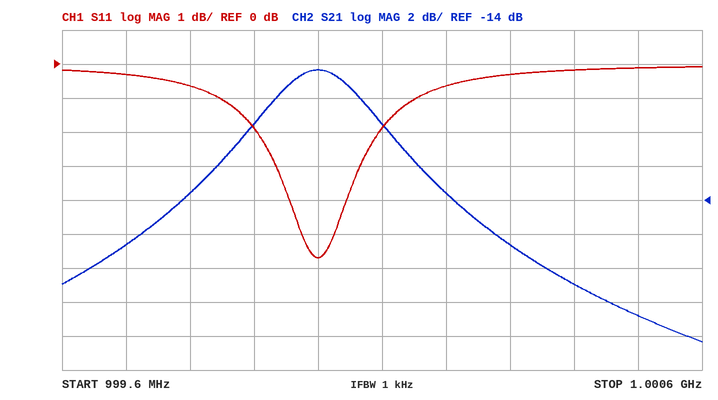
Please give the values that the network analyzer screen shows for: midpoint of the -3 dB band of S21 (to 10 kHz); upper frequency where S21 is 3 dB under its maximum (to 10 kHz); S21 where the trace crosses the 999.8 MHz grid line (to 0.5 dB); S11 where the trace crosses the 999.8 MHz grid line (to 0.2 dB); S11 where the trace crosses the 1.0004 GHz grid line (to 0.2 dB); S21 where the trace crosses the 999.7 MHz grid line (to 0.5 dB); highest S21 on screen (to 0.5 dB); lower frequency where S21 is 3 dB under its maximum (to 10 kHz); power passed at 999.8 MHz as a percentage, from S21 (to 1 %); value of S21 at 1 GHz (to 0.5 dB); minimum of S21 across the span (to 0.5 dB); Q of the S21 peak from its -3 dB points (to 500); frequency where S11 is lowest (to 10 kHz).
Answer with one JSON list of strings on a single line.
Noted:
["1.00000 GHz", "1.00010 GHz", "-13.5 dB", "-0.6 dB", "-0.2 dB", "-16.5 dB", "-6.5 dB", "999.90 MHz", "4 %", "-6.5 dB", "-22.5 dB", "5000", "1.00000 GHz"]
